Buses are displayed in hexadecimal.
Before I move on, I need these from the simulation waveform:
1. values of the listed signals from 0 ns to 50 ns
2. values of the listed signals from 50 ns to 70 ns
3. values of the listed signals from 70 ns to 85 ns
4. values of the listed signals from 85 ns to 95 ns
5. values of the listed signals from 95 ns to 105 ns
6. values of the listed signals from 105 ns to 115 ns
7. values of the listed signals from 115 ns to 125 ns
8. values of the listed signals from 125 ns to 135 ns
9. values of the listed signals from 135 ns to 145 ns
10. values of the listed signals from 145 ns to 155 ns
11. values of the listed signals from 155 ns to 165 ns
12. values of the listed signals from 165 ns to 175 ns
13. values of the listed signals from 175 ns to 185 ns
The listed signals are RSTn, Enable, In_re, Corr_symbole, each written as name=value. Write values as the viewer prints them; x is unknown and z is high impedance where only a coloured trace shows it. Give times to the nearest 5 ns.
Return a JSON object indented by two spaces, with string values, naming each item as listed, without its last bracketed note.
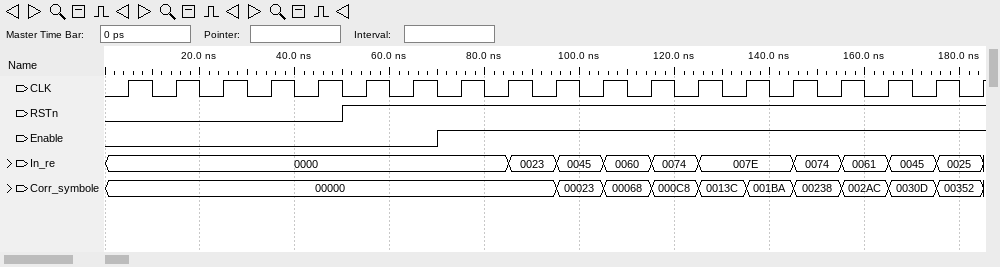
{
  "values of the listed signals from 0 ns to 50 ns": "RSTn=0, Enable=0, In_re=0000, Corr_symbole=00000",
  "values of the listed signals from 50 ns to 70 ns": "RSTn=1, Enable=0, In_re=0000, Corr_symbole=00000",
  "values of the listed signals from 70 ns to 85 ns": "RSTn=1, Enable=1, In_re=0000, Corr_symbole=00000",
  "values of the listed signals from 85 ns to 95 ns": "RSTn=1, Enable=1, In_re=0023, Corr_symbole=00000",
  "values of the listed signals from 95 ns to 105 ns": "RSTn=1, Enable=1, In_re=0045, Corr_symbole=00023",
  "values of the listed signals from 105 ns to 115 ns": "RSTn=1, Enable=1, In_re=0060, Corr_symbole=00068",
  "values of the listed signals from 115 ns to 125 ns": "RSTn=1, Enable=1, In_re=0074, Corr_symbole=000C8",
  "values of the listed signals from 125 ns to 135 ns": "RSTn=1, Enable=1, In_re=007E, Corr_symbole=0013C",
  "values of the listed signals from 135 ns to 145 ns": "RSTn=1, Enable=1, In_re=007E, Corr_symbole=001BA",
  "values of the listed signals from 145 ns to 155 ns": "RSTn=1, Enable=1, In_re=0074, Corr_symbole=00238",
  "values of the listed signals from 155 ns to 165 ns": "RSTn=1, Enable=1, In_re=0061, Corr_symbole=002AC",
  "values of the listed signals from 165 ns to 175 ns": "RSTn=1, Enable=1, In_re=0045, Corr_symbole=0030D",
  "values of the listed signals from 175 ns to 185 ns": "RSTn=1, Enable=1, In_re=0025, Corr_symbole=00352"
}
